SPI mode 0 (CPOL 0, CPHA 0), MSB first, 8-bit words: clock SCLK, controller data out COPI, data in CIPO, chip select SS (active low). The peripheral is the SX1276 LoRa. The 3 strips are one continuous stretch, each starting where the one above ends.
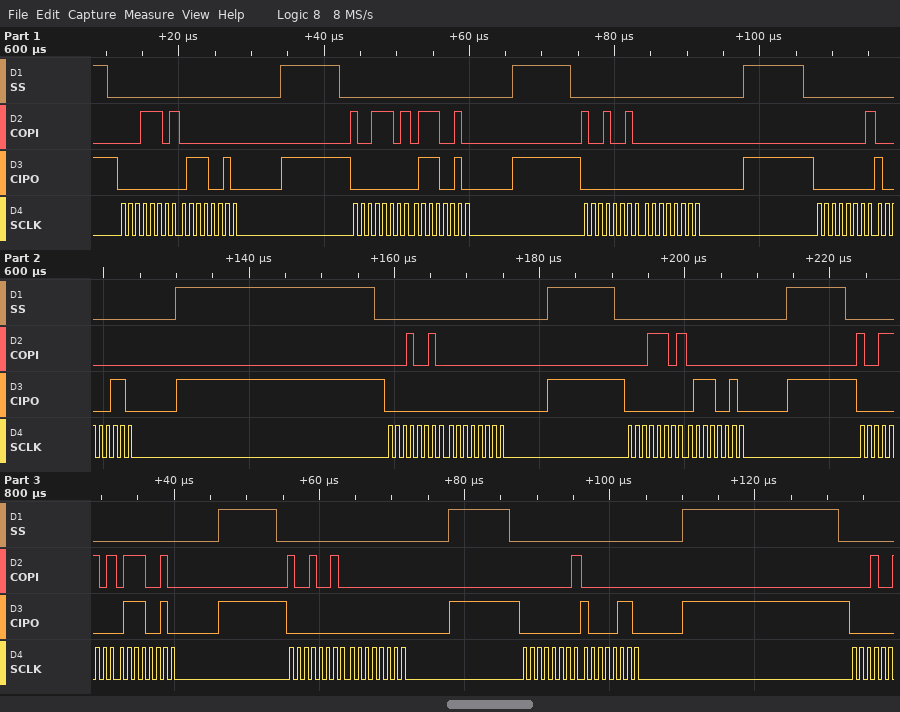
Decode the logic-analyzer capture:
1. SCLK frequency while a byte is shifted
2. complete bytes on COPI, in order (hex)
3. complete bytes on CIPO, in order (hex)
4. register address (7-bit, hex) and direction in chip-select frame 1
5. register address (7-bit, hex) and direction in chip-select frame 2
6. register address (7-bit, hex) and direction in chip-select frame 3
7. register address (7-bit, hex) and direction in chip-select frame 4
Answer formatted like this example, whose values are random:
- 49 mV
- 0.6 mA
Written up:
- 1 MHz
- 1D 00 9D 72 92 00 01 00 12 00 1D 00 9D 72 92 00 01 00
- 00 72 00 72 00 00 00 86 00 00 00 72 00 72 00 00 00 86
- 0x1D read
- 0x1D write
- 0x12 write
- 0x01 read
